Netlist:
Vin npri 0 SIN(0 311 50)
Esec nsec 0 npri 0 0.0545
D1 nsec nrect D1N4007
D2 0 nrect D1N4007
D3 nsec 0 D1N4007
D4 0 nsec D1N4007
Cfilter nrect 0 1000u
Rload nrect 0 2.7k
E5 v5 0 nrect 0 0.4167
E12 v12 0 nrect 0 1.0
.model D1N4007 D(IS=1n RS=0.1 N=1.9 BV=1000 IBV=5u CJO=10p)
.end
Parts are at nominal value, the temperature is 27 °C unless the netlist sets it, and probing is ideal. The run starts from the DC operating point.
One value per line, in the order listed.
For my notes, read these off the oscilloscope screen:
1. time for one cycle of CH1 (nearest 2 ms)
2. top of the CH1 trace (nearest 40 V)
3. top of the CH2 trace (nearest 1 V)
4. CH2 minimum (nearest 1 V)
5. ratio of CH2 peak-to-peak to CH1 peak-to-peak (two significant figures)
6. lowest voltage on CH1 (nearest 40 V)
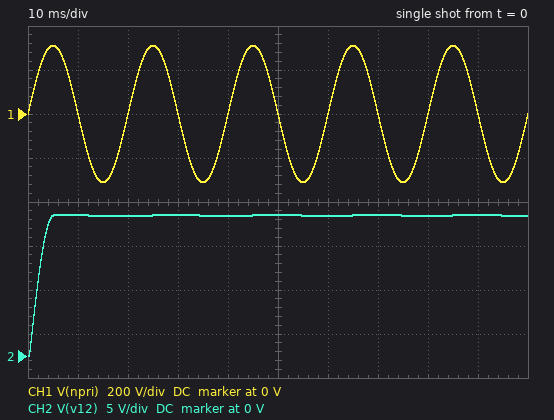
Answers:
20 ms
320 V
16 V
0 V
0.026
-320 V
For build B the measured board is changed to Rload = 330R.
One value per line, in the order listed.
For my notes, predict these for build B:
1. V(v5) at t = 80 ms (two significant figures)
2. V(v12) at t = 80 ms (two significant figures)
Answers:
6.4 V
15 V
